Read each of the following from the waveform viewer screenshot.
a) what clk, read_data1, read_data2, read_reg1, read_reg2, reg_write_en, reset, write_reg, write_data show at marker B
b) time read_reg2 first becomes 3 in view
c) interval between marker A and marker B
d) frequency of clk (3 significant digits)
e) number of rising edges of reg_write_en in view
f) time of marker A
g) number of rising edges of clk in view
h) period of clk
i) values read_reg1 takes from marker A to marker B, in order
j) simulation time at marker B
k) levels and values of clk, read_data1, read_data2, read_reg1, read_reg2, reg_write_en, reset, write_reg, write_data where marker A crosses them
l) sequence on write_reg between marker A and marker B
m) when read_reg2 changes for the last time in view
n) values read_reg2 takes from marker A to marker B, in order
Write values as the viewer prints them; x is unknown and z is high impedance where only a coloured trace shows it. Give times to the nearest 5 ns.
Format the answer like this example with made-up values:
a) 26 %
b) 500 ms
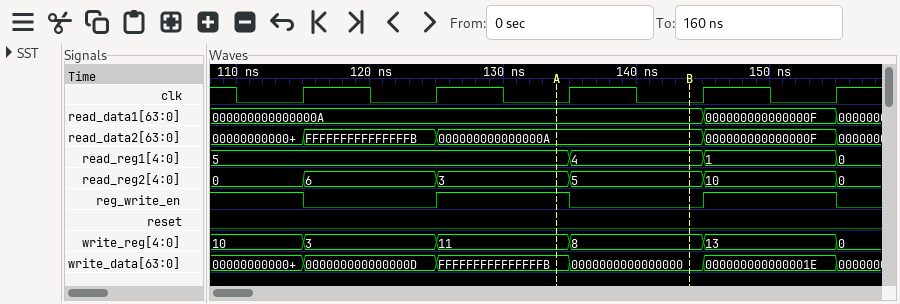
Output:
a) clk=0, read_data1=000000000000000A, read_data2=000000000000000A, read_reg1=4, read_reg2=5, reg_write_en=0, reset=0, write_reg=8, write_data=0000000000000000
b) 125 ns
c) 10 ns
d) 100 MHz
e) 2
f) 135 ns
g) 5
h) 10 ns
i) 5, 4
j) 145 ns
k) clk=0, read_data1=000000000000000A, read_data2=000000000000000A, read_reg1=5, read_reg2=3, reg_write_en=1, reset=0, write_reg=11, write_data=FFFFFFFFFFFFFFFB
l) 11, 8
m) 155 ns
n) 3, 5
